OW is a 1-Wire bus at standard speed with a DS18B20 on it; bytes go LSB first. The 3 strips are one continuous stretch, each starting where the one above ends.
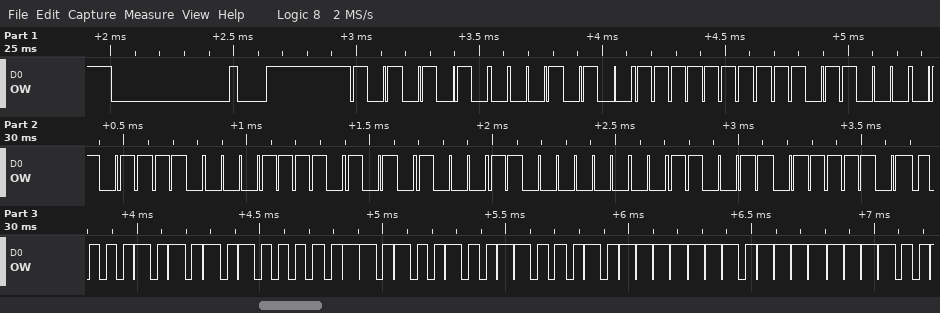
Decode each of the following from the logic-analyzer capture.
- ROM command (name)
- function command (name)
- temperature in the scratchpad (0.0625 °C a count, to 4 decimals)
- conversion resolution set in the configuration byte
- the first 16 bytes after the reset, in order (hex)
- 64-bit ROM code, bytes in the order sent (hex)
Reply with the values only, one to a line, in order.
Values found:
Match ROM
Read Scratchpad
85.0000 °C
12 bits
55 28 FF 1B 7A 78 15 03 CC BE 50 05 4B 46 7F FF
28 FF 1B 7A 78 15 03 CC
